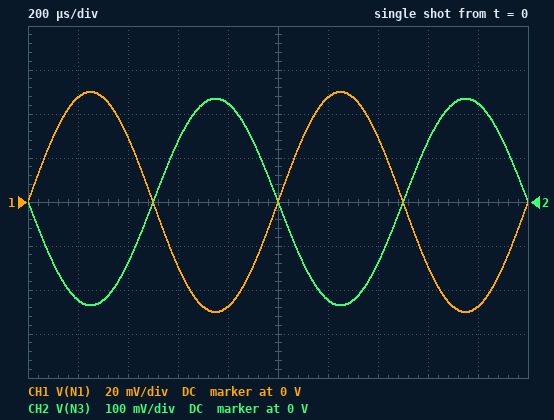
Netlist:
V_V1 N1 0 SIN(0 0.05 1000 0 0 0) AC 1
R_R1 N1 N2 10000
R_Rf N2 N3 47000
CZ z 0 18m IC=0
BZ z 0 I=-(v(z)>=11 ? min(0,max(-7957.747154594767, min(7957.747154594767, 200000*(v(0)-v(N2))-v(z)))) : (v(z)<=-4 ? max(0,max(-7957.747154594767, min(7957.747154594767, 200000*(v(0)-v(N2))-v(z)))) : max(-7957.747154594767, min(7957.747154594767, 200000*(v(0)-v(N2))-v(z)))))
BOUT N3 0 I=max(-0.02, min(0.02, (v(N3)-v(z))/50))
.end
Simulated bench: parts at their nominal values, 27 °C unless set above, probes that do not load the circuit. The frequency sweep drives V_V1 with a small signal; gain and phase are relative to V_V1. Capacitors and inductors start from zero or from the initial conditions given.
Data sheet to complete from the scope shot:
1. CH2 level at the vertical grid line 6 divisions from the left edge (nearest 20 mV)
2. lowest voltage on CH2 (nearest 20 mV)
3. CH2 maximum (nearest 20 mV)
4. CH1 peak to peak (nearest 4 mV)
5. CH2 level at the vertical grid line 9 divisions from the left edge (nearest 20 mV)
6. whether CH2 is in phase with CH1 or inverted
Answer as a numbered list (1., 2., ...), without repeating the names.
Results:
1. -220 mV
2. -240 mV
3. 240 mV
4. 100 mV
5. 220 mV
6. inverted
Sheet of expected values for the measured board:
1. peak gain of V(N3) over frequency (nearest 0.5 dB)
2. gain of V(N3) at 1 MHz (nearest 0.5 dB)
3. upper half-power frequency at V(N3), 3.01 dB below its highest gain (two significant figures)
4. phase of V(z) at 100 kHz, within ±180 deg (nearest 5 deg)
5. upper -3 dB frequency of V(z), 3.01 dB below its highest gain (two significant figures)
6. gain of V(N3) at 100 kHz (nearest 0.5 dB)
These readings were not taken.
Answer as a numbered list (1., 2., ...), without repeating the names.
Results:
1. 13.5 dB
2. 3.0 dB
3. 310 kHz
4. 160 deg
5. 310 kHz
6. 13.0 dB
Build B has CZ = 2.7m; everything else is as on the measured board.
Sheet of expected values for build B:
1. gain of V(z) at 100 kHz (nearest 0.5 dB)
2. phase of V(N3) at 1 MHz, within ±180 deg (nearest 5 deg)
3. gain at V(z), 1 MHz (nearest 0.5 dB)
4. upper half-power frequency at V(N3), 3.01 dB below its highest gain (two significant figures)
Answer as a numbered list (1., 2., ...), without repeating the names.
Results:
1. 13.5 dB
2. 155 deg
3. 12.5 dB
4. 2.1 MHz
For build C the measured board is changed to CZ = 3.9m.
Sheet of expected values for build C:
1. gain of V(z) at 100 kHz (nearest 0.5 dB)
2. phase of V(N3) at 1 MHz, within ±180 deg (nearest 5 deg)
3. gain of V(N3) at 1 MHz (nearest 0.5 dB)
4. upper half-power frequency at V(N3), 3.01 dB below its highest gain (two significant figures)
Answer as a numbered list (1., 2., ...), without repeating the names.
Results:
1. 13.5 dB
2. 145 deg
3. 11.5 dB
4. 1.4 MHz
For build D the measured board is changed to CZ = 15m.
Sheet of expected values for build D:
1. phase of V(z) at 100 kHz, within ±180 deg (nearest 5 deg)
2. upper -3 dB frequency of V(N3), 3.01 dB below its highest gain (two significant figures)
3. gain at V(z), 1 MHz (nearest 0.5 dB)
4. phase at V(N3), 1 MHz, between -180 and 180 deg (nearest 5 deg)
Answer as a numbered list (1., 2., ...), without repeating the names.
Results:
1. 165 deg
2. 370 kHz
3. 4.5 dB
4. 110 deg
